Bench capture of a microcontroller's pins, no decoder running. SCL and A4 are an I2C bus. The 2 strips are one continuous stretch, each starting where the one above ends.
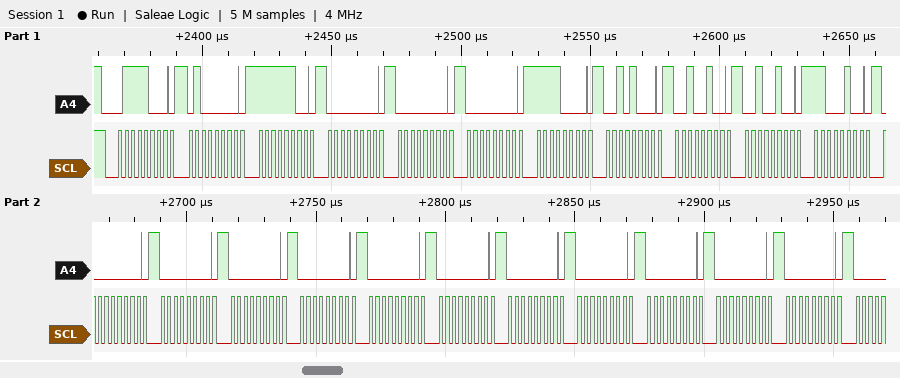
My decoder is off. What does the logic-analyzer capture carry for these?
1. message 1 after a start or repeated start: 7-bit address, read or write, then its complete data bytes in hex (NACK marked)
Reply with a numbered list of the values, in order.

1. 0x3C write: 40 FC 00 00 00 F0 28 24 24 C4 00 00 00 00 00 00 00 00 00 00 00
